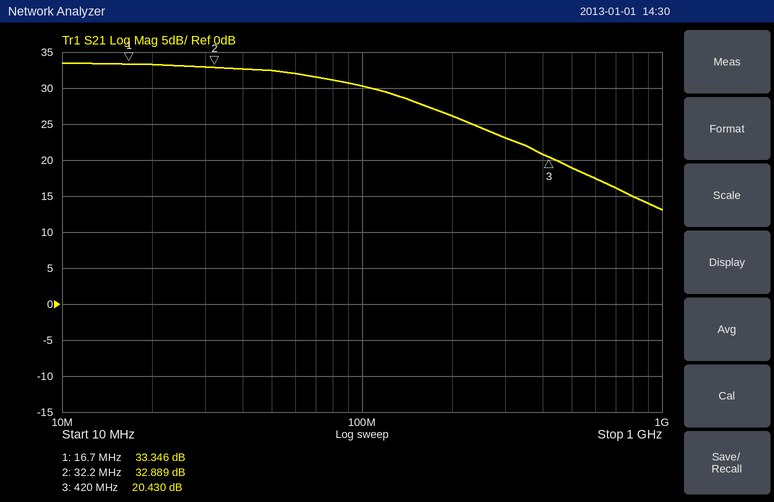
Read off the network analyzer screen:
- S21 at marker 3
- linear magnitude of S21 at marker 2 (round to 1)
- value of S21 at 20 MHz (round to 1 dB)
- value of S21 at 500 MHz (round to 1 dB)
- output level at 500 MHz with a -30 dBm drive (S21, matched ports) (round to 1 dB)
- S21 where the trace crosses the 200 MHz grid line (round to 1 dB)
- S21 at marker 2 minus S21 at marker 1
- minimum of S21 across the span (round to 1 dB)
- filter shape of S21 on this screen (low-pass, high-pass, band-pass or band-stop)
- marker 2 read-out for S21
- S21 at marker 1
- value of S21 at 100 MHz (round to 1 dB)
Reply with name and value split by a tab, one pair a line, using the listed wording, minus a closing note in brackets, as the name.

S21 at marker 3	20.430 dB
linear magnitude of S21 at marker 2	44
value of S21 at 20 MHz	33 dB
value of S21 at 500 MHz	19 dB
output level at 500 MHz with a -30 dBm drive (S21, matched ports)	-11 dBm
S21 where the trace crosses the 200 MHz grid line	26 dB
S21 at marker 2 minus S21 at marker 1	-0.457 dB
minimum of S21 across the span	13 dB
filter shape of S21 on this screen	low-pass
marker 2 read-out for S21	32.889 dB
S21 at marker 1	33.346 dB
value of S21 at 100 MHz	30 dB
